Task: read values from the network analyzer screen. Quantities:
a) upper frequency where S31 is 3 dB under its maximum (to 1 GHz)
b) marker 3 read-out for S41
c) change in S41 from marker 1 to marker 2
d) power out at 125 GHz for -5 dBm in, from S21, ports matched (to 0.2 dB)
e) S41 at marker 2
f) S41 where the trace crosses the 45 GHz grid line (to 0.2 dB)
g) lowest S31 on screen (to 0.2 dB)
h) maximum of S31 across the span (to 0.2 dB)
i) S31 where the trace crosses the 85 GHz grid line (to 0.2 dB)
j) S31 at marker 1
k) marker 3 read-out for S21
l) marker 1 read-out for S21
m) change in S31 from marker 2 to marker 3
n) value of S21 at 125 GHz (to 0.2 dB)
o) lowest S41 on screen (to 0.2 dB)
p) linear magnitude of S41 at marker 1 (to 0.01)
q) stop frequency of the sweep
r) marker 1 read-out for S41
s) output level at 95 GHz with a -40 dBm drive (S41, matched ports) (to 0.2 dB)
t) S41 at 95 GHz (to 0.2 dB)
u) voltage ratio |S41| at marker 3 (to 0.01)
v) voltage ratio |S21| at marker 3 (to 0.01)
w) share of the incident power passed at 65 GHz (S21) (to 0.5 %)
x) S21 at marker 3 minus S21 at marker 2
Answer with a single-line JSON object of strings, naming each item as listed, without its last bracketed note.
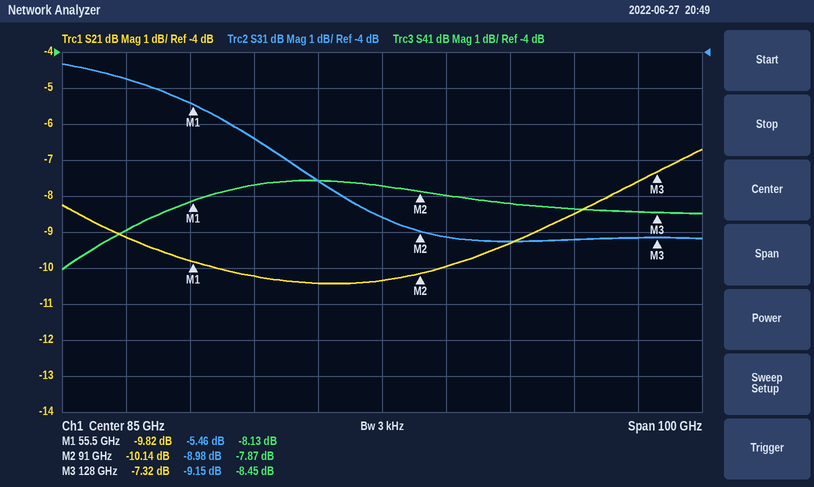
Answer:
{"upper frequency where S31 is 3 dB under its maximum": "73 GHz", "marker 3 read-out for S41": "-8.45 dB", "change in S41 from marker 1 to marker 2": "0.26 dB", "power out at 125 GHz for -5 dBm in, from S21, ports matched": "-12.6 dBm", "S41 at marker 2": "-7.87 dB", "S41 where the trace crosses the 45 GHz grid line": "-9.0 dB", "lowest S31 on screen": "-9.2 dB", "maximum of S31 across the span": "-4.4 dB", "S31 where the trace crosses the 85 GHz grid line": "-8.6 dB", "S31 at marker 1": "-5.46 dB", "marker 3 read-out for S21": "-7.32 dB", "marker 1 read-out for S21": "-9.82 dB", "change in S31 from marker 2 to marker 3": "-0.17 dB", "value of S21 at 125 GHz": "-7.6 dB", "lowest S41 on screen": "-10.0 dB", "linear magnitude of S41 at marker 1": "0.39", "stop frequency of the sweep": "135 GHz", "marker 1 read-out for S41": "-8.13 dB", "output level at 95 GHz with a -40 dBm drive (S41, matched ports)": "-48.0 dBm", "S41 at 95 GHz": "-8.0 dB", "voltage ratio |S41| at marker 3": "0.38", "voltage ratio |S21| at marker 3": "0.43", "share of the incident power passed at 65 GHz (S21)": "9.5 %", "S21 at marker 3 minus S21 at marker 2": "2.82 dB"}
